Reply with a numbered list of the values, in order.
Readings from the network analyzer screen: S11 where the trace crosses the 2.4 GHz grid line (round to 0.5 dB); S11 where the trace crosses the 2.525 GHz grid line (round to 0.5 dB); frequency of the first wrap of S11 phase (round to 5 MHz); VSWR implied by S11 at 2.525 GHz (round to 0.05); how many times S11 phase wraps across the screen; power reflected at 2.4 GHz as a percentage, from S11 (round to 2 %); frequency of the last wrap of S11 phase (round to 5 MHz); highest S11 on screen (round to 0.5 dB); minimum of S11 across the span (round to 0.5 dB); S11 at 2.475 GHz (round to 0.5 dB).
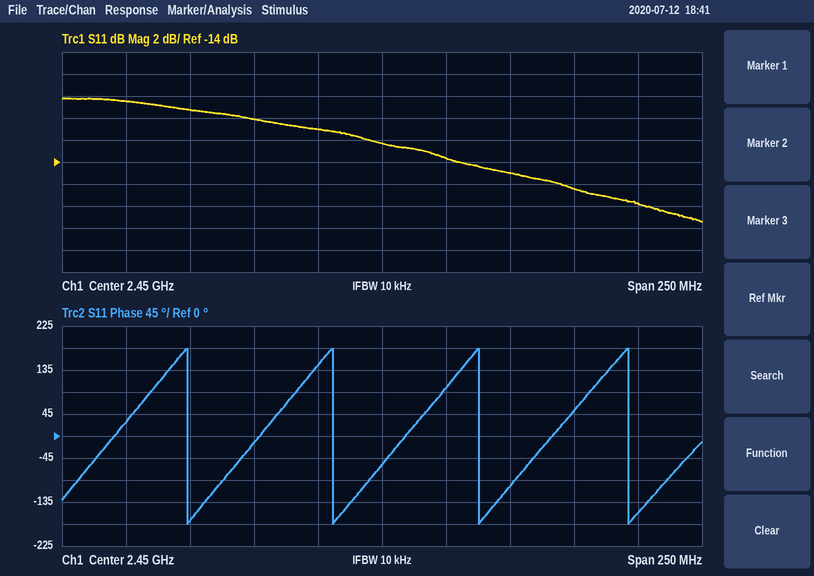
1. -10.0 dB
2. -16.5 dB
3. 2.375 GHz
4. 1.35
5. 4
6. 10 %
7. 2.545 GHz
8. -8.0 dB
9. -19.5 dB
10. -13.5 dB
